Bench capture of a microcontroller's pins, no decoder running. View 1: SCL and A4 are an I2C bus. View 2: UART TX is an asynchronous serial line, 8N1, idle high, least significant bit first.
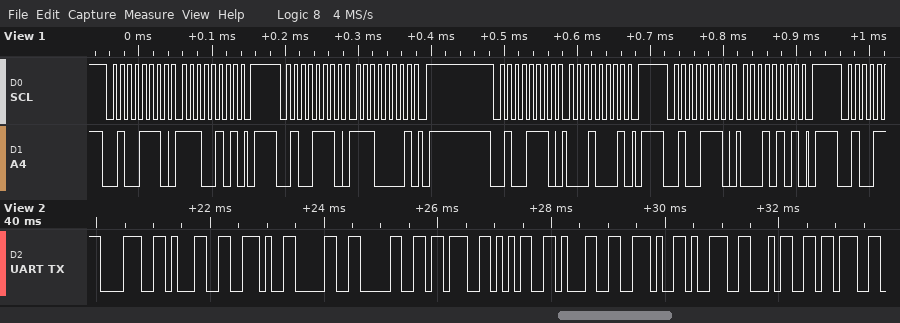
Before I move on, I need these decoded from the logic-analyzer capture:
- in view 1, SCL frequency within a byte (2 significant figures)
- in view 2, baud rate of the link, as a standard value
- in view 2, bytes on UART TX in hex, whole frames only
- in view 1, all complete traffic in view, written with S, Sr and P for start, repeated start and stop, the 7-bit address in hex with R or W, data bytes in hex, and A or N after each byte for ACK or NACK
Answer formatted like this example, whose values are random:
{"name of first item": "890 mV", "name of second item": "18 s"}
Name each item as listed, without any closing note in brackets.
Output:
{"in view 1, SCL frequency within a byte": "100 kHz", "in view 2, baud rate of the link, as a standard value": "9600 baud", "in view 2, bytes on UART TX in hex, whole frames only": "0x38 0x31 0x2E 0x30 0x30 0x3B 0x35 0x31 0x2E 0x39 0x34 0x3B", "in view 1, all complete traffic in view, written with S, Sr and P for start, repeated start and stop, the 7-bit address in hex with R or W, data bytes in hex, and A or N after each byte for ACK or NACK": "S 27W A E5 A P S 27W A E1 A P S 27W A 11 A P S 27W A 15 A P"}
